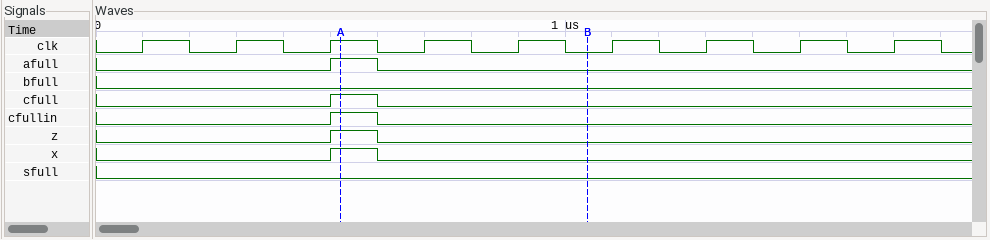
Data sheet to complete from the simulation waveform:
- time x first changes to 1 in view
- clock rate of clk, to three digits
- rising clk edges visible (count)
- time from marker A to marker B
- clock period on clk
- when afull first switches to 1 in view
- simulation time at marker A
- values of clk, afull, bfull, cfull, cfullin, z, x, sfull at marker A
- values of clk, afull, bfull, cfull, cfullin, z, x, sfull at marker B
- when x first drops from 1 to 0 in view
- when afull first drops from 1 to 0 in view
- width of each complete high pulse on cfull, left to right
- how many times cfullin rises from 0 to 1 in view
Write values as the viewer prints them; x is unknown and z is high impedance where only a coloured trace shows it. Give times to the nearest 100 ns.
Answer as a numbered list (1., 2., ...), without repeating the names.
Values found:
1. 500 ns
2. 5.00 MHz
3. 9
4. 500 ns
5. 200 ns
6. 500 ns
7. 500 ns
8. clk=1, afull=1, bfull=0, cfull=1, cfullin=1, z=1, x=1, sfull=0
9. clk=0, afull=0, bfull=0, cfull=0, cfullin=0, z=0, x=0, sfull=0
10. 600 ns
11. 600 ns
12. 100 ns
13. 1
